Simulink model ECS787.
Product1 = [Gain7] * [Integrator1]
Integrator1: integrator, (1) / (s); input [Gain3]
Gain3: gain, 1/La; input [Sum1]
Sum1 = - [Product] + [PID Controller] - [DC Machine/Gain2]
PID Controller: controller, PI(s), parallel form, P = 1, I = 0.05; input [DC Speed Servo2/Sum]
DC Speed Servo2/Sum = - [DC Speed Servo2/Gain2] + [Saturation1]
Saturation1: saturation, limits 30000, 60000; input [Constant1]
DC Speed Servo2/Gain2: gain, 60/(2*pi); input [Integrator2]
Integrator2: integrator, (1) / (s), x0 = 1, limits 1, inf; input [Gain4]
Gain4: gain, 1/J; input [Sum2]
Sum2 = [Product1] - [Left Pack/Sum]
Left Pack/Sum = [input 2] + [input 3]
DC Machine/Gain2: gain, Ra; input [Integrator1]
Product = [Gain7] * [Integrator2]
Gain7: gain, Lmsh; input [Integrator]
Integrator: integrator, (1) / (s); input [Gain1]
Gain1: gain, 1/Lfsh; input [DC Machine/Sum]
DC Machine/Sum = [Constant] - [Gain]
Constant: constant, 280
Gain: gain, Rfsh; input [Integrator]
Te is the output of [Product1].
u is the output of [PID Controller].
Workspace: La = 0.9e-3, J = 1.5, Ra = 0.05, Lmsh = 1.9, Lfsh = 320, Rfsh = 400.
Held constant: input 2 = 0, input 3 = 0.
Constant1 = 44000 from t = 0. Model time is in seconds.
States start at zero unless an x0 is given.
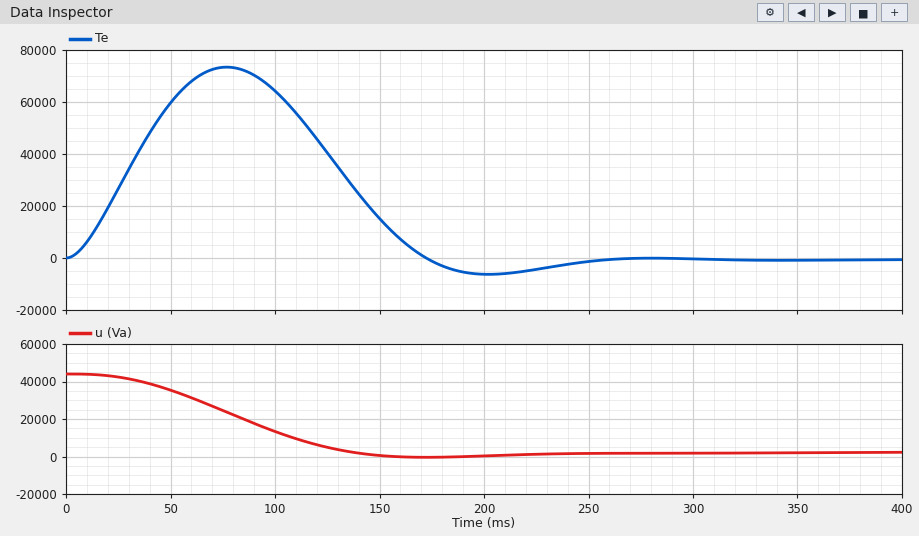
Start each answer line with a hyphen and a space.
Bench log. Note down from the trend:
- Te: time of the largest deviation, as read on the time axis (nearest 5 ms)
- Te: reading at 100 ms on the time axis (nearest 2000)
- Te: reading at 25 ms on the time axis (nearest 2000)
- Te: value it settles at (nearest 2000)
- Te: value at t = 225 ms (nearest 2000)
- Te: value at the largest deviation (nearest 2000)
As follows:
- 75 ms
- 64000
- 26000
- 0
- -4000
- 74000
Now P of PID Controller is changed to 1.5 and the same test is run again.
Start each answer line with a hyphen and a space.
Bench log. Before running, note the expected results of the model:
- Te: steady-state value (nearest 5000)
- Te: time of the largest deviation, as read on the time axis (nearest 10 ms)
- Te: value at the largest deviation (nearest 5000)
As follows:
- 0
- 70 ms
- 95000
